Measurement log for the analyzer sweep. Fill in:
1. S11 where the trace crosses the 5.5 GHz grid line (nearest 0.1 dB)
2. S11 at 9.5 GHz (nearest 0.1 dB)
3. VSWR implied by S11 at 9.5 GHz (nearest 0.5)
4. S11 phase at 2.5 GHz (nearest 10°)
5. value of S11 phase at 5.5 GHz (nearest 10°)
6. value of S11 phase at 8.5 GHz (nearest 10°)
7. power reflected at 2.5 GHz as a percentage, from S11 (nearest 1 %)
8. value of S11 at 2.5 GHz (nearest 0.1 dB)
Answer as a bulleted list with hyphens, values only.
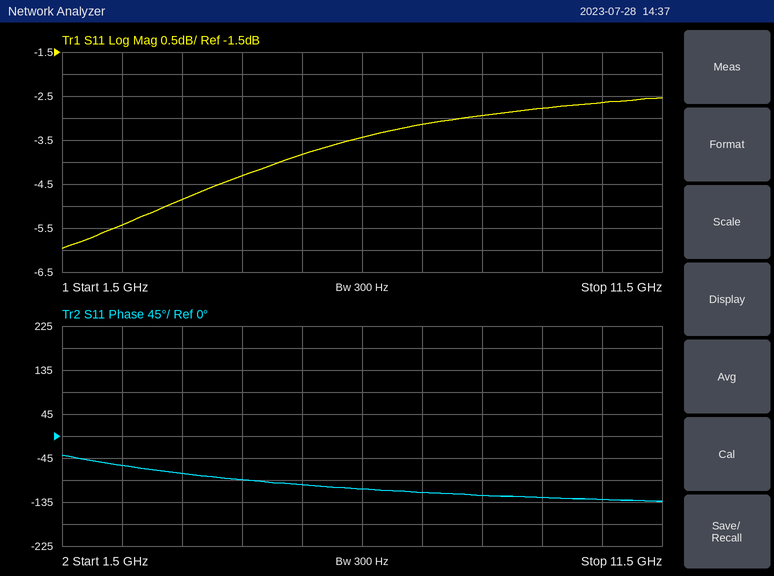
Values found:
- -3.8 dB
- -2.8 dB
- 6.5
- -60°
- -100°
- -120°
- 29 %
- -5.4 dB
